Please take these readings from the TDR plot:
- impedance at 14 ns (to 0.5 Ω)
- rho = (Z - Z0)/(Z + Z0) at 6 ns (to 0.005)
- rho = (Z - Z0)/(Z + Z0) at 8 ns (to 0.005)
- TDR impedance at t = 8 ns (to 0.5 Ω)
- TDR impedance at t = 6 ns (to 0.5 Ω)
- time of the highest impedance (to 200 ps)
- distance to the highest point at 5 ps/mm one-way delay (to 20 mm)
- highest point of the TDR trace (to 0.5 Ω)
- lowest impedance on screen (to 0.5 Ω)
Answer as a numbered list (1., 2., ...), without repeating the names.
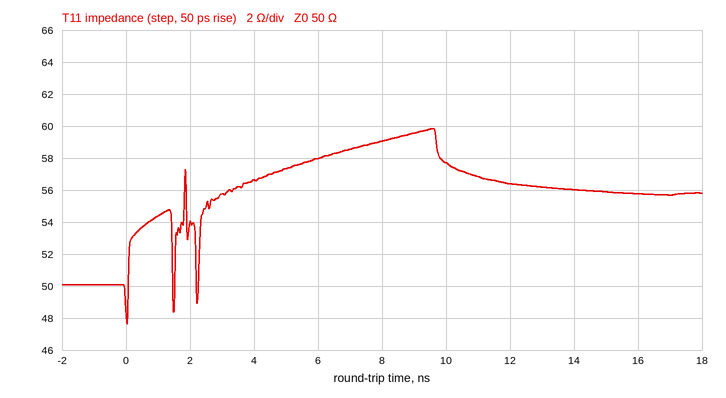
1. 56.0 Ω
2. +0.075
3. +0.085
4. 59.0 Ω
5. 58.0 Ω
6. 9.6 ns
7. 960 mm
8. 60.0 Ω
9. 47.5 Ω
